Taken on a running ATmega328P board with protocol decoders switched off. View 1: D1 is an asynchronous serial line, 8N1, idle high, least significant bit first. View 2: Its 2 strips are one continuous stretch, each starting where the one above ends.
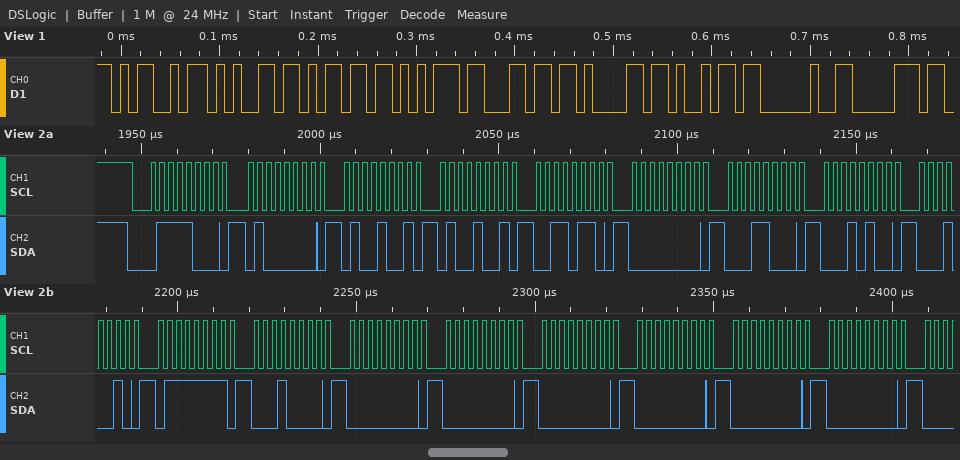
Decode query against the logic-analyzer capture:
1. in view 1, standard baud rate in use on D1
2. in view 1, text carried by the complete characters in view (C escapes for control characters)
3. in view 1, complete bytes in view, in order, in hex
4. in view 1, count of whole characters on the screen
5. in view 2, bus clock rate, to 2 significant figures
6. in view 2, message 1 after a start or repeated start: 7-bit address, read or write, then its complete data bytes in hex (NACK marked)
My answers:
115200 baud
"Memulai p"
0x4D 0x65 0x6D 0x75 0x6C 0x61 0x69 0x20 0x70
9
400 kHz
0x3C write: 40 49 49 36 00 18 14 12 7F 10 00 00 00 00 00 00
